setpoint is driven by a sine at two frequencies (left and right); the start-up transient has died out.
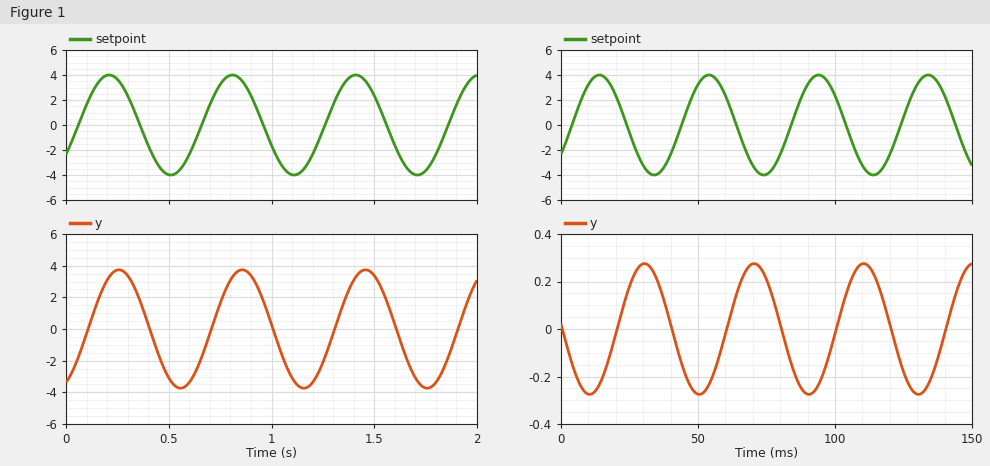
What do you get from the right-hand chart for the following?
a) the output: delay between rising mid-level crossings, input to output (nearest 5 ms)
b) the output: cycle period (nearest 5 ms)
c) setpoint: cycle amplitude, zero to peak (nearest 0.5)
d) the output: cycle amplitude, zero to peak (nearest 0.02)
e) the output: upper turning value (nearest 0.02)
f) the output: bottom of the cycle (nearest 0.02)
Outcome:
15 ms
40 ms
4.0
0.28
0.28
-0.28
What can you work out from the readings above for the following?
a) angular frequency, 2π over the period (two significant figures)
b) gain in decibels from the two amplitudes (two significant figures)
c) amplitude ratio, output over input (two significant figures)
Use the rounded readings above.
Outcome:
0.16 rad/ms
-23 dB
0.070
